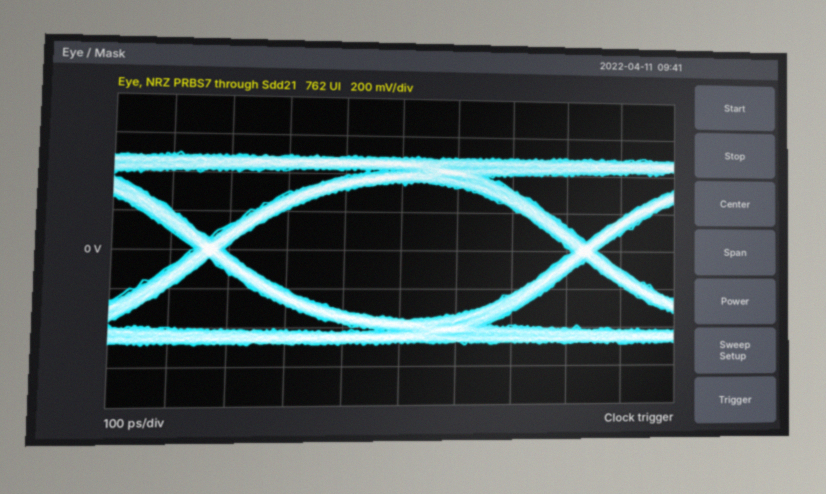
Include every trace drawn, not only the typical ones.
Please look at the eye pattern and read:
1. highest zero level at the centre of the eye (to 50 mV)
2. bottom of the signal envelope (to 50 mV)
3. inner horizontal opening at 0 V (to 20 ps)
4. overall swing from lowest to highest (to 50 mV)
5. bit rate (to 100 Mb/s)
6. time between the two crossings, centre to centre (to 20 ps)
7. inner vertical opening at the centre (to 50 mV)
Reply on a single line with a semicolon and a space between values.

-350 mV; -500 mV; 620 ps; 1.00 V; 1.5 Gb/s; 660 ps; 700 mV
